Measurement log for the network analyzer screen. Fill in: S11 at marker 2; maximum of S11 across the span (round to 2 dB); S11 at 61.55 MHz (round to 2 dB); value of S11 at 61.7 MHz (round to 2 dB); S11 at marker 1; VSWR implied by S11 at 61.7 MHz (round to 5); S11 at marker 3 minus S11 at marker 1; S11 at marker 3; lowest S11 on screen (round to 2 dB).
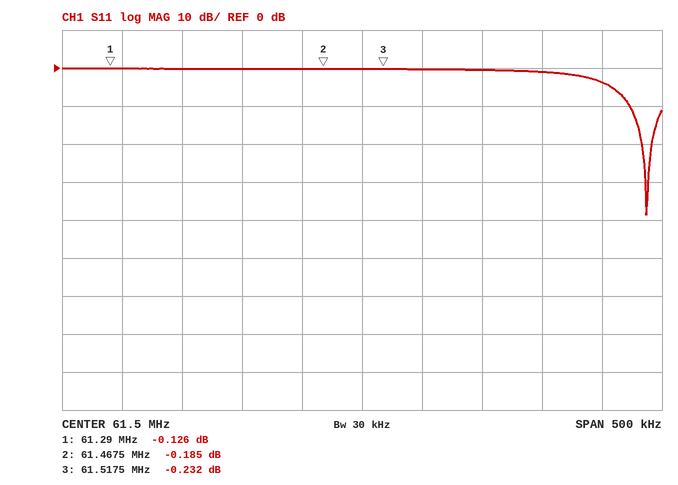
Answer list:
-0.185 dB
0 dB
0 dB
-4 dB
-0.126 dB
5
-0.106 dB
-0.232 dB
-38 dB
